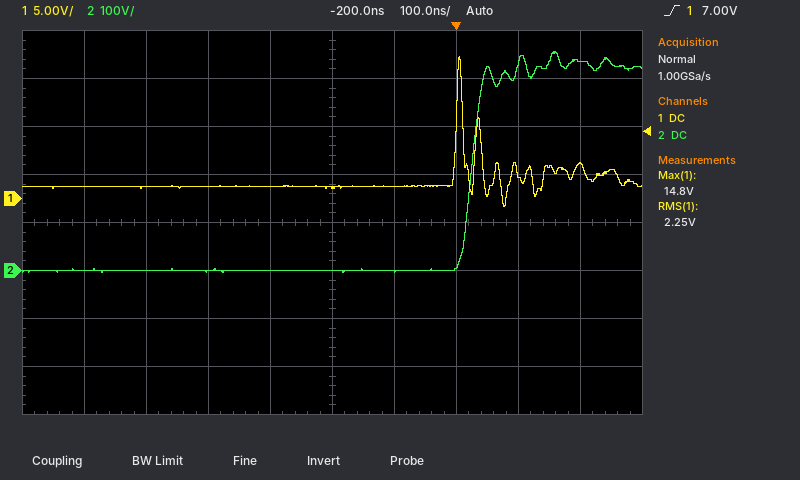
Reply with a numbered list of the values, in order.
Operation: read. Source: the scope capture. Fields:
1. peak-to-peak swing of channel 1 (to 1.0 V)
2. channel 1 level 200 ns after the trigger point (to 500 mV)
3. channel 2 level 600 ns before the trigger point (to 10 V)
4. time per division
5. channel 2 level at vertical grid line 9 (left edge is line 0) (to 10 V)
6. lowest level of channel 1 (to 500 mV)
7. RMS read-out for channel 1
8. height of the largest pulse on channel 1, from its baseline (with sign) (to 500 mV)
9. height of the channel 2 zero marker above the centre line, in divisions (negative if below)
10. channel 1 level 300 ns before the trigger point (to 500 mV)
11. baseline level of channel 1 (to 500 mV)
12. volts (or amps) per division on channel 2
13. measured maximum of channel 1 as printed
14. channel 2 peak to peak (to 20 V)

1. 16.0 V
2. 3.5 V
3. 0 V
4. 100 ns
5. 440 V
6. -1.0 V
7. 2.25 V
8. +13.5 V
9. -1.0 div
10. 1.0 V
11. 1.0 V
12. 100 V
13. 14.8 V
14. 460 V
